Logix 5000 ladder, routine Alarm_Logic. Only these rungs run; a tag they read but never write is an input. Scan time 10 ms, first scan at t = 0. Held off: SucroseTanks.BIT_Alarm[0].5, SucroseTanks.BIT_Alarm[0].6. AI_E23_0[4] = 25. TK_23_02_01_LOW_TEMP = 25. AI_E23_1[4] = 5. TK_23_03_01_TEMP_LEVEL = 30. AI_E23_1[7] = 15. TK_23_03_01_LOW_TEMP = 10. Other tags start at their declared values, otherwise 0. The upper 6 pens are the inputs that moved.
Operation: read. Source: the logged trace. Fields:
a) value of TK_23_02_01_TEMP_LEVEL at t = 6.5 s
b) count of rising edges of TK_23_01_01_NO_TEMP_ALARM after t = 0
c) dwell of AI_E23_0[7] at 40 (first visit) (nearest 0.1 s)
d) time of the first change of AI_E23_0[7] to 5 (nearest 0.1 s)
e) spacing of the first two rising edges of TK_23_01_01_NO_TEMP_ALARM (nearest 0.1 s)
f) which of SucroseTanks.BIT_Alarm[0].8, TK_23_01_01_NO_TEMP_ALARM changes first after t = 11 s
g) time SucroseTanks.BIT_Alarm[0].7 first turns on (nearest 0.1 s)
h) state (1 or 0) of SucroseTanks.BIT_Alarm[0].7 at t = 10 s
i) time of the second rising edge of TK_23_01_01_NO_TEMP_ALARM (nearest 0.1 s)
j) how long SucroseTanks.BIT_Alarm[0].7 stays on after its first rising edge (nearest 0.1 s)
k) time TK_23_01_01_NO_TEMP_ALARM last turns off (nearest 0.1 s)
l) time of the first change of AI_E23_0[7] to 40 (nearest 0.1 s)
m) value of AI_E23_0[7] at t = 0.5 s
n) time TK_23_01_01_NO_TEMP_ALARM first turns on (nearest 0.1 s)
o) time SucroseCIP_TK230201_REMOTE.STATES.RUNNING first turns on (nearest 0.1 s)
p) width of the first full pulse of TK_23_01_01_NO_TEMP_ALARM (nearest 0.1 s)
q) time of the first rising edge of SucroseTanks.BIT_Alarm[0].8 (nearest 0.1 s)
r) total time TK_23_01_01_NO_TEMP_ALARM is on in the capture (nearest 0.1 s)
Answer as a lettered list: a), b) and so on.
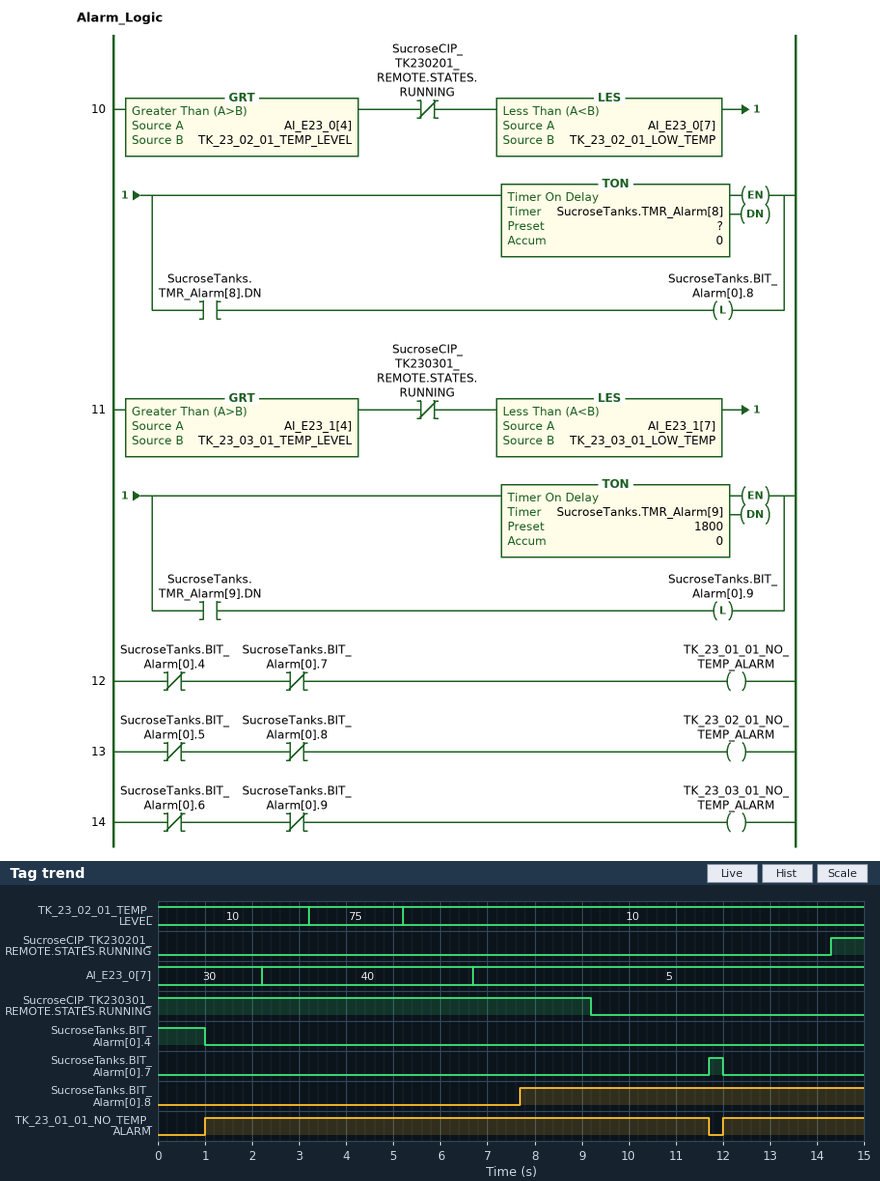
a) 10
b) 2
c) 4.5 s
d) 6.7 s
e) 11.0 s
f) TK_23_01_01_NO_TEMP_ALARM
g) 11.7 s
h) 0
i) 12.0 s
j) 0.3 s
k) 11.7 s
l) 2.2 s
m) 30
n) 1.0 s
o) 14.3 s
p) 10.7 s
q) 7.7 s
r) 13.7 s
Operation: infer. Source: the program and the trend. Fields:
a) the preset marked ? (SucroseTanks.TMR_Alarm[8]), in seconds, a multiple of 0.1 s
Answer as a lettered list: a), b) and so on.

a) 1.0 s
